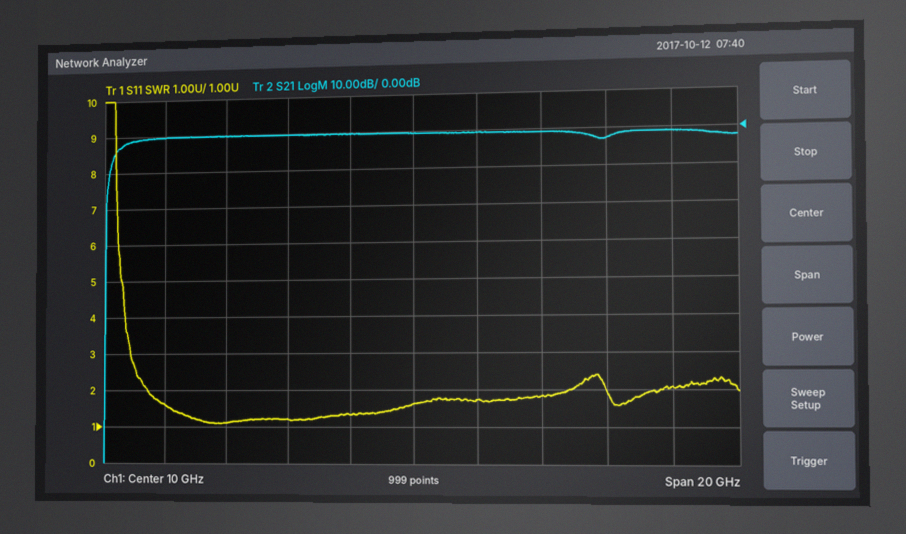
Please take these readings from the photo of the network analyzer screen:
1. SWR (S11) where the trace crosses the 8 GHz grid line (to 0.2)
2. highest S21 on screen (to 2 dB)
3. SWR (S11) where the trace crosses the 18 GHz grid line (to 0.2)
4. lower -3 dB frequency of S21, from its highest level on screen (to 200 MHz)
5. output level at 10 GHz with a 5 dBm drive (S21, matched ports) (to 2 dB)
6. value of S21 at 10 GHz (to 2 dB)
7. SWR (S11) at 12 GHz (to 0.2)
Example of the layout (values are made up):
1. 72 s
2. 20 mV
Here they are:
1. 1.4
2. 0 dB
3. 2.0
4. 400 MHz
5. 4 dBm
6. 0 dB
7. 1.8
